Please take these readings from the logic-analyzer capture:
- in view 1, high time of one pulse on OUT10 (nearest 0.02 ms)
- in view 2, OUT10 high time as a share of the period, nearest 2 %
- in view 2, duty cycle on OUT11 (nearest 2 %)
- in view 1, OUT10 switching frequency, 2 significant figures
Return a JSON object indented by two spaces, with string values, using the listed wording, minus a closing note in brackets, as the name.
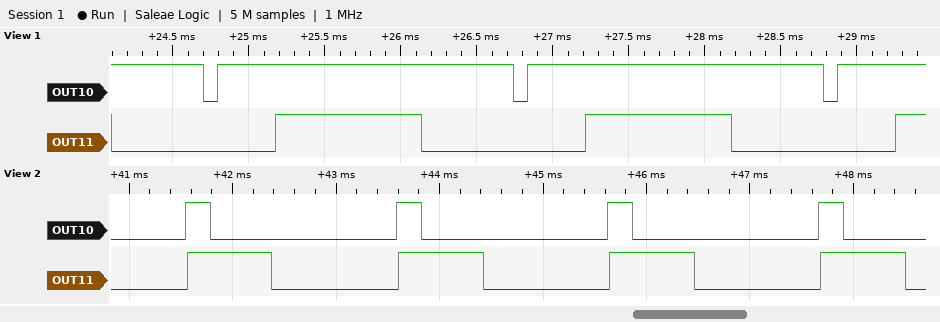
{
  "in view 1, high time of one pulse on OUT10": "1.94 ms",
  "in view 2, OUT10 high time as a share of the period, nearest 2 %": "12 %",
  "in view 2, duty cycle on OUT11": "40 %",
  "in view 1, OUT10 switching frequency, 2 significant figures": "490 Hz"
}
